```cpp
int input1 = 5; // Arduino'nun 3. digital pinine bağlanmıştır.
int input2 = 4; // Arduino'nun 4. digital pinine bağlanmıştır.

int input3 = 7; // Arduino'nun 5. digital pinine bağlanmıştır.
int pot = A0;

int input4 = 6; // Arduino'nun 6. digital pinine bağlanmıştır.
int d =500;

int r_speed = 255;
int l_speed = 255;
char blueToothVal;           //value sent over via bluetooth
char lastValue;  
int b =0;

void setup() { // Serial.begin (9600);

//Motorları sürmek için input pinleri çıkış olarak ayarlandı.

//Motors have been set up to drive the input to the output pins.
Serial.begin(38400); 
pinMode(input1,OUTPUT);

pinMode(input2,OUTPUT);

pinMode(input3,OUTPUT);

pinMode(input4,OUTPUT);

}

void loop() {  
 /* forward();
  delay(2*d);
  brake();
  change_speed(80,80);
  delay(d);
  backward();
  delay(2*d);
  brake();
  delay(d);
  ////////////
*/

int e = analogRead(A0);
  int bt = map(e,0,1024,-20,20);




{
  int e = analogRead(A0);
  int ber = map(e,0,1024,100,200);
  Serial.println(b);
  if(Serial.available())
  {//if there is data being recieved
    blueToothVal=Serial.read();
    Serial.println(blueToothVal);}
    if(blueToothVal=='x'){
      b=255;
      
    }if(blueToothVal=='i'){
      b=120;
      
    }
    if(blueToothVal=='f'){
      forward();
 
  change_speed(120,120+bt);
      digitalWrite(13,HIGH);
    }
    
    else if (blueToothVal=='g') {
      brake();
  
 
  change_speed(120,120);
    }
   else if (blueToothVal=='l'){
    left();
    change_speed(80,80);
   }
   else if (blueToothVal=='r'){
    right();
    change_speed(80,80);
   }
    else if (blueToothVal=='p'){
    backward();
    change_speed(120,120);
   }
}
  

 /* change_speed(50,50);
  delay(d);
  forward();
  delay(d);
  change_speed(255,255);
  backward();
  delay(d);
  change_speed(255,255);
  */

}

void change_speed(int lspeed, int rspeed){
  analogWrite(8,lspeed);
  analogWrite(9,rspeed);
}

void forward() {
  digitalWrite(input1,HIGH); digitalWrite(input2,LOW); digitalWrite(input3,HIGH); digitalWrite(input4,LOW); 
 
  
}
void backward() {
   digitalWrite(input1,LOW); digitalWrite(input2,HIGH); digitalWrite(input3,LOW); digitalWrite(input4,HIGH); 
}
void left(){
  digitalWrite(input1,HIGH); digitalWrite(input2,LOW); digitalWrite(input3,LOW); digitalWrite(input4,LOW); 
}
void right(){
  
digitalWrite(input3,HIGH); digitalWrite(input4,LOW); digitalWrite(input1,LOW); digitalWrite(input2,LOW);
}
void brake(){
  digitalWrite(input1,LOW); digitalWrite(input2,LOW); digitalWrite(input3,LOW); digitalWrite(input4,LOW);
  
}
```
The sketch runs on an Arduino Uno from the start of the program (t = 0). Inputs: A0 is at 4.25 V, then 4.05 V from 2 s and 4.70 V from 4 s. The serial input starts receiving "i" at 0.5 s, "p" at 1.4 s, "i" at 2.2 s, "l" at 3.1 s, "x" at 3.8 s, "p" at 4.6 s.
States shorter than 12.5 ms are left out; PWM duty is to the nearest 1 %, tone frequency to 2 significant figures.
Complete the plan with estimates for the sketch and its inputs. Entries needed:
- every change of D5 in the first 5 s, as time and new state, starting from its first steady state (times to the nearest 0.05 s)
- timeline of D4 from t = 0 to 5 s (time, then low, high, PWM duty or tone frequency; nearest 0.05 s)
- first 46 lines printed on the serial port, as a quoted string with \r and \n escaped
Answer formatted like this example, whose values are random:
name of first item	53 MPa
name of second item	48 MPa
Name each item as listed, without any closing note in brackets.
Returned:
every change of D5 in the first 5 s, as time and new state, starting from its first steady state	0 s low; 3.1 s high; 4.6 s low
timeline of D4 from t = 0 to 5 s	0 s low; 1.4 s high; 3.1 s low; 4.6 s high
first 46 lines printed on the serial port, as a quoted string with \r and \n escaped	"0\r\n0\r\n0\r\n0\r\n0\r\n0\r\n0\r\n0\r\n0\r\n0\r\n0\r\n0\r\n0\r\n0\r\n0\r\n0\r\n0\r\n0\r\n0\r\n0\r\n0\r\n0\r\n0\r\n0\r\n0\r\n0\r\n0\r\n0\r\n0\r\n0\r\n0\r\n0\r\n0\r\n0\r\n0\r\n0\r\n0\r\n0\r\n0\r\n0\r\n0\r\n0\r\n0\r\n0\r\n0\r\n0\r\n"
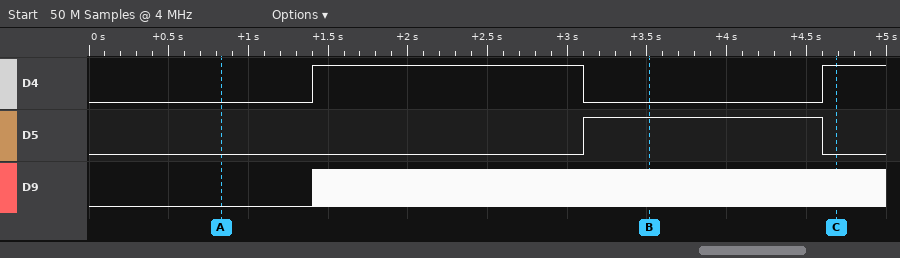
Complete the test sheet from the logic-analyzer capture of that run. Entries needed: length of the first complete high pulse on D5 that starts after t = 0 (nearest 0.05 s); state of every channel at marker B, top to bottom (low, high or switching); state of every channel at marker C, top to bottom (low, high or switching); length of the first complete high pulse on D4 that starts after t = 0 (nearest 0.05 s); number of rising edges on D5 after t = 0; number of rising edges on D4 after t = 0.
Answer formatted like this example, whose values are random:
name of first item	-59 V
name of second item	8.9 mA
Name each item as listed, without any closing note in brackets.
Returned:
length of the first complete high pulse on D5 that starts after t = 0	1.50 s
state of every channel at marker B, top to bottom	D4 low, D5 high, D9 switching
state of every channel at marker C, top to bottom	D4 high, D5 low, D9 switching
length of the first complete high pulse on D4 that starts after t = 0	1.70 s
number of rising edges on D5 after t = 0	1
number of rising edges on D4 after t = 0	2
